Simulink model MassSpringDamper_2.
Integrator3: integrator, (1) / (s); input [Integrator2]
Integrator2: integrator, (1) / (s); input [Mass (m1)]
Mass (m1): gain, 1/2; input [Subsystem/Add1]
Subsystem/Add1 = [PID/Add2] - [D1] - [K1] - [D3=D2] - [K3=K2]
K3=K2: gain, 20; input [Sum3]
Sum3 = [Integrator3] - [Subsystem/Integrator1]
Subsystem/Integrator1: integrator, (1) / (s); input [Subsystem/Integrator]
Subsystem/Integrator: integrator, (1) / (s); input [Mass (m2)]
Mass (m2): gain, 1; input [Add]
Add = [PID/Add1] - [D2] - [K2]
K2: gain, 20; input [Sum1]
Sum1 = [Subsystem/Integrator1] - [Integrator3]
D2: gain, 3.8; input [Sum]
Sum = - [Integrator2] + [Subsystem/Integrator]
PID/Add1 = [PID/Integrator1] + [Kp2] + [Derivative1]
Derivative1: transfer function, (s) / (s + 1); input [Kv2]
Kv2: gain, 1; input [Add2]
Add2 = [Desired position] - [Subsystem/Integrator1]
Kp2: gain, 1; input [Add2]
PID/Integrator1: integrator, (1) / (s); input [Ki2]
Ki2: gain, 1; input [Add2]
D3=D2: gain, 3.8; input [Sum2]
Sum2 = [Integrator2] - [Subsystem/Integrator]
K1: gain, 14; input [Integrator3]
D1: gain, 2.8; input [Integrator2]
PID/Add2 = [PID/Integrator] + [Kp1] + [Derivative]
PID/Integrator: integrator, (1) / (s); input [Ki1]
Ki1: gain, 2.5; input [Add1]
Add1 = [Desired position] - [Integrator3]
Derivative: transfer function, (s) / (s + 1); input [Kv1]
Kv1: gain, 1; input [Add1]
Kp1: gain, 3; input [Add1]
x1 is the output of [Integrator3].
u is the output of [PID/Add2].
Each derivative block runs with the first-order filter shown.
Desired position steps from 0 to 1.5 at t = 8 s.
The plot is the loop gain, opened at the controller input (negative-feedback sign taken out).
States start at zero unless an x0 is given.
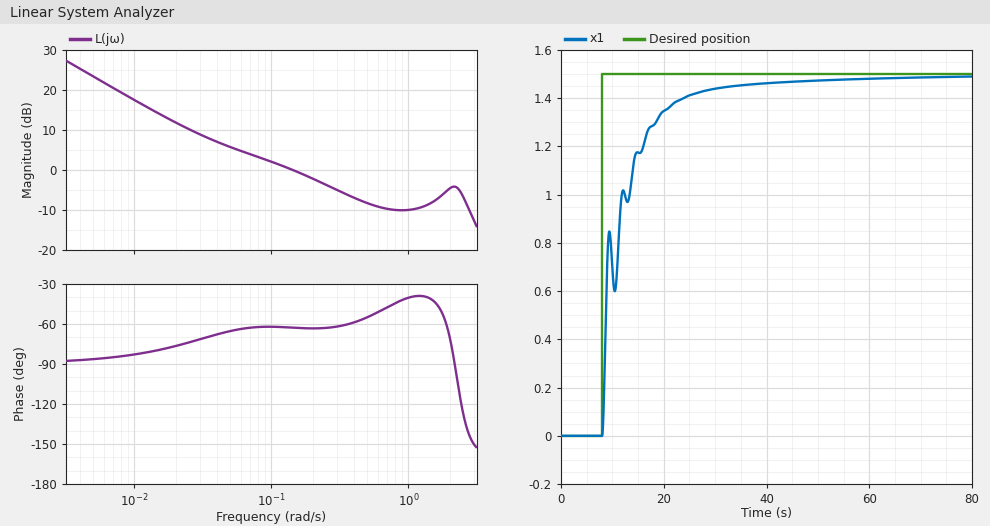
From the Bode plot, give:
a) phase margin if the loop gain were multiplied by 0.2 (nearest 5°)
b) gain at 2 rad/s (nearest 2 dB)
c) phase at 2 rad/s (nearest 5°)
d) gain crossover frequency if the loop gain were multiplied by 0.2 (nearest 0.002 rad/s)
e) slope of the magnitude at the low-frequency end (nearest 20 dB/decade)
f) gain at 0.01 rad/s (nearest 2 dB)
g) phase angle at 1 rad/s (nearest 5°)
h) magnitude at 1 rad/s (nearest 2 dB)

100°
-4 dB
-70°
0.016 rad/s
-20 dB/decade
18 dB
-40°
-10 dB
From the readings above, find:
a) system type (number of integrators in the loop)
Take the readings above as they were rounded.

1
